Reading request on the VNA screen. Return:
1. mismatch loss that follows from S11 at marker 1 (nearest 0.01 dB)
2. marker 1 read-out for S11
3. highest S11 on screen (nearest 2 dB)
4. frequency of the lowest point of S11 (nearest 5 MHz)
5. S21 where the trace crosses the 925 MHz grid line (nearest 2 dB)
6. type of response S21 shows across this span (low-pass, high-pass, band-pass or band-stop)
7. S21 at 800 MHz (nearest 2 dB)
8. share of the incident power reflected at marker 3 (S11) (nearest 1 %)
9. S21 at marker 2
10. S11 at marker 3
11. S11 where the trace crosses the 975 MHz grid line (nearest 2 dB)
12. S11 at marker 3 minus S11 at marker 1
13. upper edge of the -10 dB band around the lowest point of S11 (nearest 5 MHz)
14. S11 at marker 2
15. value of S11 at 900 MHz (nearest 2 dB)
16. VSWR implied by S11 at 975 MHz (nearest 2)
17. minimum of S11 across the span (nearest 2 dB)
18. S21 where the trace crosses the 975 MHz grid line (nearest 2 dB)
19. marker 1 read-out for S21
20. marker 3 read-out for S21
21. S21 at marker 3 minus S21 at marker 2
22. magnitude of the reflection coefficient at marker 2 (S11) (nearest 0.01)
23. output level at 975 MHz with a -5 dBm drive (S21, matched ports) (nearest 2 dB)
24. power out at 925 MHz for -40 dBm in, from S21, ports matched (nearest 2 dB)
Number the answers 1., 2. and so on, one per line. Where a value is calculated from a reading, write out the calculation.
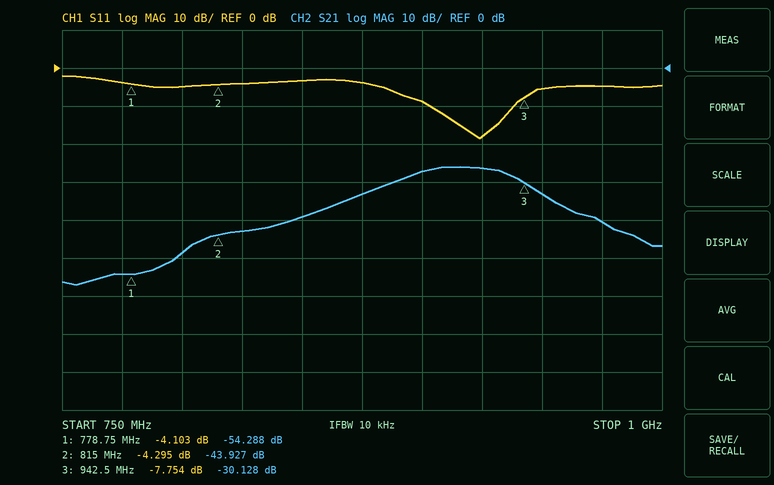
1. −10 log10(1 − 10^(-4.103/10)) ≈ 2.14 dB
2. -4.103 dB
3. -2 dB
4. 925 MHz
5. -26 dB
6. band-pass
7. -48 dB
8. 10^(-7.754/10) ≈ 17 %
9. -43.927 dB
10. -7.754 dB
11. -4 dB
12. -7.754 − (-4.103) = -3.651 dB
13. 940 MHz
14. -4.295 dB
15. -8 dB
16. |Γ| = 10^(-4/20) = 0.6310; VSWR = (1 + 0.6310)/(1 − 0.6310) ≈ 4
17. -18 dB
18. -40 dB
19. -54.288 dB
20. -30.128 dB
21. -30.128 − (-43.927) = 13.799 dB
22. 10^(-4.295/20) ≈ 0.61
23. -5 dBm + (-40 dB) = -46 dBm
24. -40 dBm + (-26 dB) = -66 dBm
